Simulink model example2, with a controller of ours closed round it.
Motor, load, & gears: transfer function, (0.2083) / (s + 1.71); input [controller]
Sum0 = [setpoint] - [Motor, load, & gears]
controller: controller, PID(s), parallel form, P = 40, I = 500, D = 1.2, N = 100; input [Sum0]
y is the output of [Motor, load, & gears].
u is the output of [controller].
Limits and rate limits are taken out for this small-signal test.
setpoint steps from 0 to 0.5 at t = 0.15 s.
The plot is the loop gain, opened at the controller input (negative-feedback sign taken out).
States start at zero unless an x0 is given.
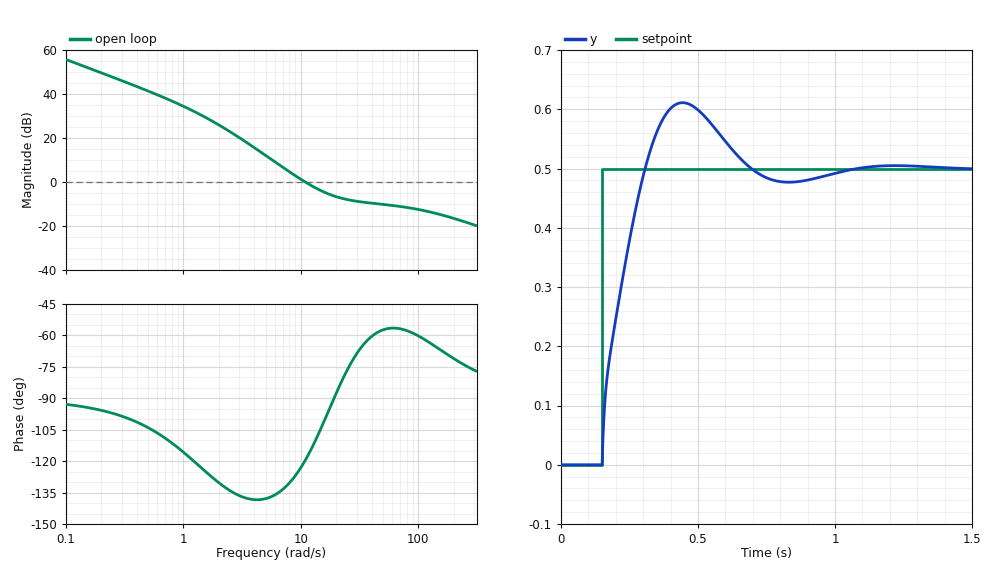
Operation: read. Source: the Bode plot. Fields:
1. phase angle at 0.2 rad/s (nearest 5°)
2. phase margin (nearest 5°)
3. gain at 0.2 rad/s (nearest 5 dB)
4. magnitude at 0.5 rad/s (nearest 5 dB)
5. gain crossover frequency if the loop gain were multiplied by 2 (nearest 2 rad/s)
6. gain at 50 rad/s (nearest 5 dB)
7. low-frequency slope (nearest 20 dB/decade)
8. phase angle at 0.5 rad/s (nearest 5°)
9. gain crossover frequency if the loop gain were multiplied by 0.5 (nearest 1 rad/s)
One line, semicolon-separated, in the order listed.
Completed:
-95°; 60°; 50 dB; 40 dB; 18 rad/s; -10 dB; -20 dB/decade; -105°; 7 rad/s
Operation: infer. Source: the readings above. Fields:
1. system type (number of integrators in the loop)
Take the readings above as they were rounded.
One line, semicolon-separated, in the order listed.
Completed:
1
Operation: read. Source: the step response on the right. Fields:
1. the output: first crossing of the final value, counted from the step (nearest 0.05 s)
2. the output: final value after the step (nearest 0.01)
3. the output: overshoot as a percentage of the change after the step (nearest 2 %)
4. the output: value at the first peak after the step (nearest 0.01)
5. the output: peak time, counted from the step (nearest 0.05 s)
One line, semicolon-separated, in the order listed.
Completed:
0.15 s; 0.50; 22 %; 0.61; 0.30 s
